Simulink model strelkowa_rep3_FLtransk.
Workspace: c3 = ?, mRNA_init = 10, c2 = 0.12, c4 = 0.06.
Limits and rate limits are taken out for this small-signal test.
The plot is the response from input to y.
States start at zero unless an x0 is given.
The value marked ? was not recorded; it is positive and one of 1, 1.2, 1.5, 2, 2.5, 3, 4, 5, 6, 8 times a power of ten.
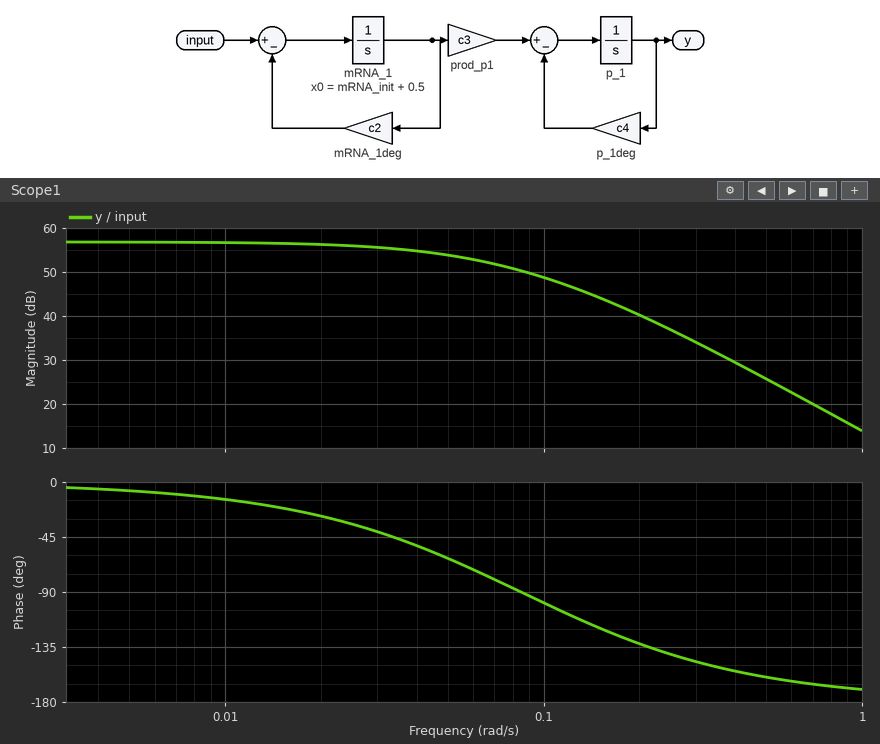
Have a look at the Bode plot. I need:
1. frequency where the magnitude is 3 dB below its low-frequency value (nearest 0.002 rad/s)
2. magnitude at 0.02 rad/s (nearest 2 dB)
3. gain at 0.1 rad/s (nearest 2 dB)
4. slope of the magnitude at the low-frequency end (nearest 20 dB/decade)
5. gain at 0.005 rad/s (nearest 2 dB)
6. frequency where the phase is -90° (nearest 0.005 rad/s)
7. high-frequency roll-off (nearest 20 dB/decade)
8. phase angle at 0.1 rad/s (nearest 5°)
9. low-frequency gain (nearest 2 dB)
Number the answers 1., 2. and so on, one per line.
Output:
1. 0.050 rad/s
2. 56 dB
3. 48 dB
4. 0 dB/decade
5. 56 dB
6. 0.085 rad/s
7. -40 dB/decade
8. -100°
9. 56 dB
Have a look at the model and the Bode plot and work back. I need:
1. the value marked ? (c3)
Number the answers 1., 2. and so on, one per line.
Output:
1. 5
